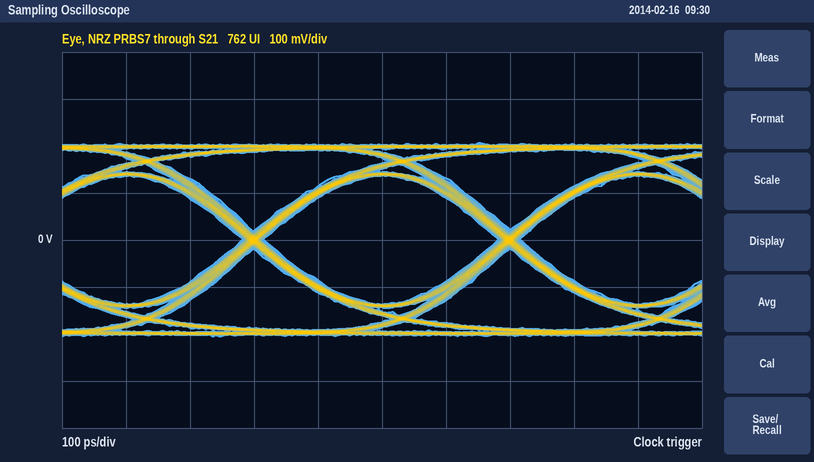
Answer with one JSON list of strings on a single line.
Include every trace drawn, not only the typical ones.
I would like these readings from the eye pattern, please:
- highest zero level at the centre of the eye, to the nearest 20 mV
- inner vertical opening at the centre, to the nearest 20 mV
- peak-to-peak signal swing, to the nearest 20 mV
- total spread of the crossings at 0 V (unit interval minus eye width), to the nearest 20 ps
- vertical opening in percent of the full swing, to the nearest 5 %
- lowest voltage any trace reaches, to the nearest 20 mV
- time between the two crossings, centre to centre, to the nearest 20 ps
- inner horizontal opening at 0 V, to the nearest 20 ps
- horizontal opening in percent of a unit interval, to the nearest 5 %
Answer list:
["-140 mV", "280 mV", "420 mV", "40 ps", "65 %", "-200 mV", "400 ps", "360 ps", "90 %"]
